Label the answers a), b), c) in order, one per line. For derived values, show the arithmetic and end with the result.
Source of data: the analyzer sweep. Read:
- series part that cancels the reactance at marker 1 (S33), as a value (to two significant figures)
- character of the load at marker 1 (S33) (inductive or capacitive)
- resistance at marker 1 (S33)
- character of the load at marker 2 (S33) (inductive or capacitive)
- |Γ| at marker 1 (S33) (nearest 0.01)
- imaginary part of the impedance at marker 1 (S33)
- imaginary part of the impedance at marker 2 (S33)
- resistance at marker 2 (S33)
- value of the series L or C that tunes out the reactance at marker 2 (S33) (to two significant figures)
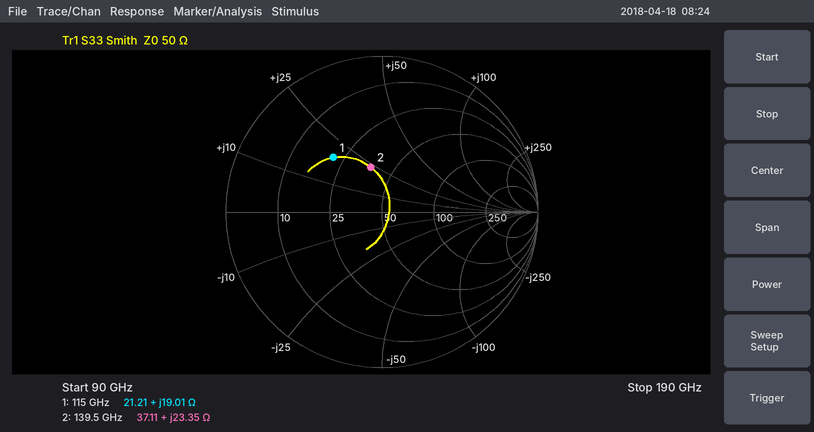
a) C = 1/(2π × 115 GHz × 19.01 Ω) ≈ 73 fF
b) inductive
c) 21.21 Ω
d) inductive
e) 0.47
f) +19.01 Ω
g) +23.35 Ω
h) 37.11 Ω
i) C = 1/(2π × 139.5 GHz × 23.35 Ω) ≈ 49 fF
